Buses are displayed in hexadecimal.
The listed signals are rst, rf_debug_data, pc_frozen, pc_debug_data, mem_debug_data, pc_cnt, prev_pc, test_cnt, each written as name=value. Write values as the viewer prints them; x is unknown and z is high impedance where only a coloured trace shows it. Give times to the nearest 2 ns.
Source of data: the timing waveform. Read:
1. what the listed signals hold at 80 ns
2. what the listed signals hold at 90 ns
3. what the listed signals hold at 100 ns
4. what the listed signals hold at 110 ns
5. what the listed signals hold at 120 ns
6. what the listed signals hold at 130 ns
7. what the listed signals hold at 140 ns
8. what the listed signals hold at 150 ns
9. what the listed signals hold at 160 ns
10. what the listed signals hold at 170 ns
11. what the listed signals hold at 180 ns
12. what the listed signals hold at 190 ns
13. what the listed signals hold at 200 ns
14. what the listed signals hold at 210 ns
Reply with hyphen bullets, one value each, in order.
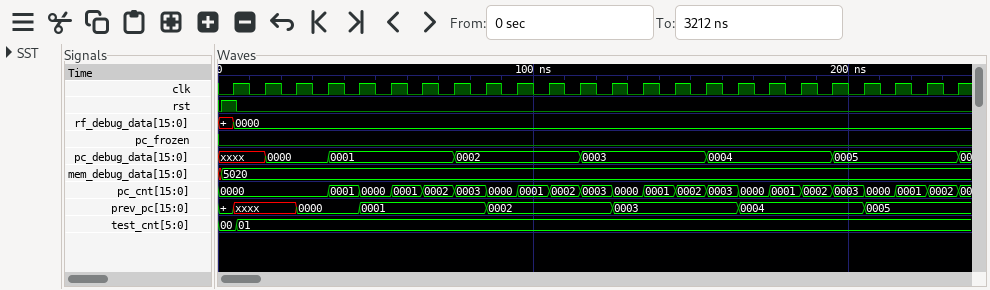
- rst=0, rf_debug_data=0000, pc_frozen=0, pc_debug_data=0002, mem_debug_data=5020, pc_cnt=0003, prev_pc=0001, test_cnt=01
- rst=0, rf_debug_data=0000, pc_frozen=0, pc_debug_data=0002, mem_debug_data=5020, pc_cnt=0000, prev_pc=0002, test_cnt=01
- rst=0, rf_debug_data=0000, pc_frozen=0, pc_debug_data=0002, mem_debug_data=5020, pc_cnt=0001, prev_pc=0002, test_cnt=01
- rst=0, rf_debug_data=0000, pc_frozen=0, pc_debug_data=0002, mem_debug_data=5020, pc_cnt=0002, prev_pc=0002, test_cnt=01
- rst=0, rf_debug_data=0000, pc_frozen=0, pc_debug_data=0003, mem_debug_data=5020, pc_cnt=0003, prev_pc=0002, test_cnt=01
- rst=0, rf_debug_data=0000, pc_frozen=0, pc_debug_data=0003, mem_debug_data=5020, pc_cnt=0000, prev_pc=0003, test_cnt=01
- rst=0, rf_debug_data=0000, pc_frozen=0, pc_debug_data=0003, mem_debug_data=5020, pc_cnt=0001, prev_pc=0003, test_cnt=01
- rst=0, rf_debug_data=0000, pc_frozen=0, pc_debug_data=0003, mem_debug_data=5020, pc_cnt=0002, prev_pc=0003, test_cnt=01
- rst=0, rf_debug_data=0000, pc_frozen=0, pc_debug_data=0004, mem_debug_data=5020, pc_cnt=0003, prev_pc=0003, test_cnt=01
- rst=0, rf_debug_data=0000, pc_frozen=0, pc_debug_data=0004, mem_debug_data=5020, pc_cnt=0000, prev_pc=0004, test_cnt=01
- rst=0, rf_debug_data=0000, pc_frozen=0, pc_debug_data=0004, mem_debug_data=5020, pc_cnt=0001, prev_pc=0004, test_cnt=01
- rst=0, rf_debug_data=0000, pc_frozen=0, pc_debug_data=0004, mem_debug_data=5020, pc_cnt=0002, prev_pc=0004, test_cnt=01
- rst=0, rf_debug_data=0000, pc_frozen=0, pc_debug_data=0005, mem_debug_data=5020, pc_cnt=0003, prev_pc=0004, test_cnt=01
- rst=0, rf_debug_data=0000, pc_frozen=0, pc_debug_data=0005, mem_debug_data=5020, pc_cnt=0000, prev_pc=0005, test_cnt=01
